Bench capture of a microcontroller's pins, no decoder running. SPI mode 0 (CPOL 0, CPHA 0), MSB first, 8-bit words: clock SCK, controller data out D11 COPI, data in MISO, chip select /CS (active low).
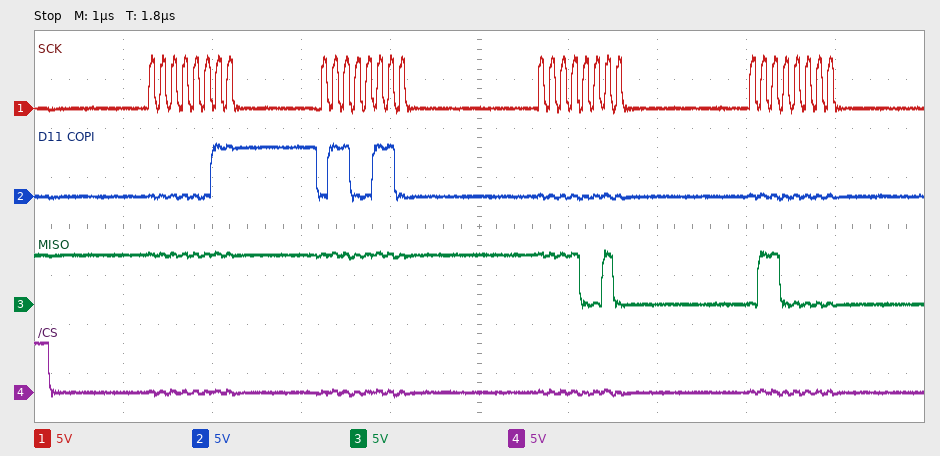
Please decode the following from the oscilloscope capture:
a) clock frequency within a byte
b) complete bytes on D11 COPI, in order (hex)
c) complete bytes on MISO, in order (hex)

8 MHz
03 66 00 00
FF FF F2 60
